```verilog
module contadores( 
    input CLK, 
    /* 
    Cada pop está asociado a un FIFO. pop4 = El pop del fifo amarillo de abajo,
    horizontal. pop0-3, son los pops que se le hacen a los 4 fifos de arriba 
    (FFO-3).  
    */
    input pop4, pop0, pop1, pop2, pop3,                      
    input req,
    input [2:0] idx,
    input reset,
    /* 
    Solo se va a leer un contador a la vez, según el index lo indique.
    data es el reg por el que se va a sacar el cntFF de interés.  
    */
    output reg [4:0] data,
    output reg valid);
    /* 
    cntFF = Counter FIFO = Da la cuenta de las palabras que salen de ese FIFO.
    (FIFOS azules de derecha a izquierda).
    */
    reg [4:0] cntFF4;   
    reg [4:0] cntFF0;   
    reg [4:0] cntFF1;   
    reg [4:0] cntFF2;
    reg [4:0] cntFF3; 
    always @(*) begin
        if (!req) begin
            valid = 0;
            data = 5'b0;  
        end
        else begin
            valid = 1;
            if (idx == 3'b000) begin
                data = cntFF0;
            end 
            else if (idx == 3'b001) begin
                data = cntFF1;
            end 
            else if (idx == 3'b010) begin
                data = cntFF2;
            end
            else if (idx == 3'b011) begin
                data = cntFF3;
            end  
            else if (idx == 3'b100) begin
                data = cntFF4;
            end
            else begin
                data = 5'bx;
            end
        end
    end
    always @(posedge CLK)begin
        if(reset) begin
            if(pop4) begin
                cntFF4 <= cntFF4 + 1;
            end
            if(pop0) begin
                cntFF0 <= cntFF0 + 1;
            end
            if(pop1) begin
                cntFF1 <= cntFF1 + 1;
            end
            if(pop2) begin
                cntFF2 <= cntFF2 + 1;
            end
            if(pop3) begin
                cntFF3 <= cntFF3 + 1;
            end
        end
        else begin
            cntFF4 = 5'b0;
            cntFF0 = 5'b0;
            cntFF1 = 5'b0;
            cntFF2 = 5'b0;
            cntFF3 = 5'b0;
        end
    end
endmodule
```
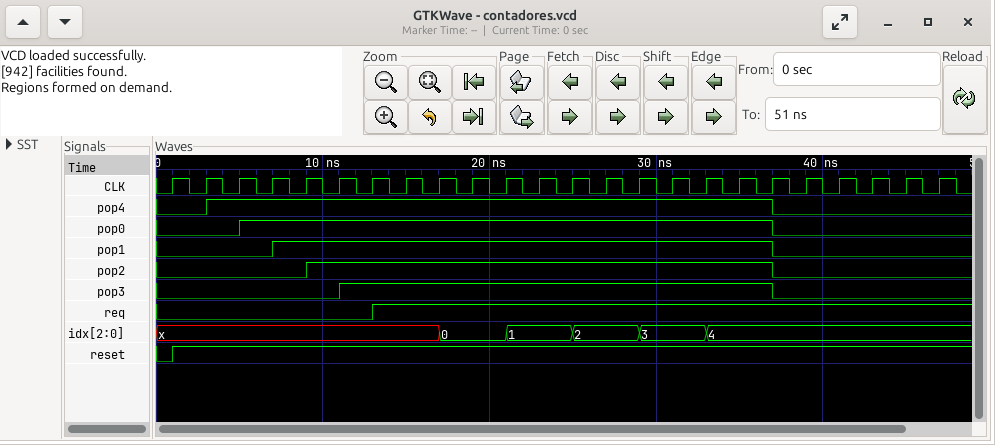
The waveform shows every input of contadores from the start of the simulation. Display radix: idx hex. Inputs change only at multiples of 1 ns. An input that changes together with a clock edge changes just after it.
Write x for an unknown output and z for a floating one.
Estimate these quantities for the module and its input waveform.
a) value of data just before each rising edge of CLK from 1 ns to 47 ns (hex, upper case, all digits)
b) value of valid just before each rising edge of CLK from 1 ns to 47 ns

00, 00, 00, 00, 00, 00, 00, x, x, 06, 07, 07, 08, 08, 09, 09, 0A, 0F, 10, 11, 11, 11, 11, 11
0 0 0 0 0 0 0 1 1 1 1 1 1 1 1 1 1 1 1 1 1 1 1 1
